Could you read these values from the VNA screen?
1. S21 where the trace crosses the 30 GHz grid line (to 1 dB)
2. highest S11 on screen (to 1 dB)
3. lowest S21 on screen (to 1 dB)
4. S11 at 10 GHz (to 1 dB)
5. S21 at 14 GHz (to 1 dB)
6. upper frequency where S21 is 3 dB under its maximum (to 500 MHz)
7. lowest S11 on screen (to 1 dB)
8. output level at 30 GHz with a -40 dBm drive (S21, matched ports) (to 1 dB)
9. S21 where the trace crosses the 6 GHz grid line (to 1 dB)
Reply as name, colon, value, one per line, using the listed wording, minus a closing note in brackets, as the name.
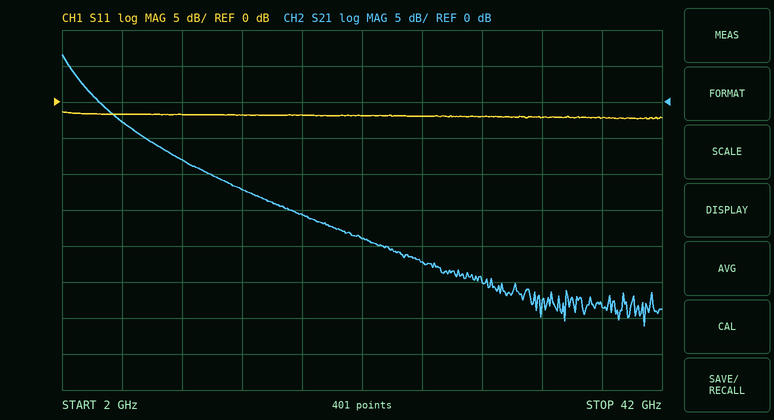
S21 where the trace crosses the 30 GHz grid line: -25 dB
highest S11 on screen: -1 dB
lowest S21 on screen: -31 dB
S11 at 10 GHz: -2 dB
S21 at 14 GHz: -12 dB
upper frequency where S21 is 3 dB under its maximum: 3.0 GHz
lowest S11 on screen: -2 dB
output level at 30 GHz with a -40 dBm drive (S21, matched ports): -65 dBm
S21 where the trace crosses the 6 GHz grid line: -3 dB
